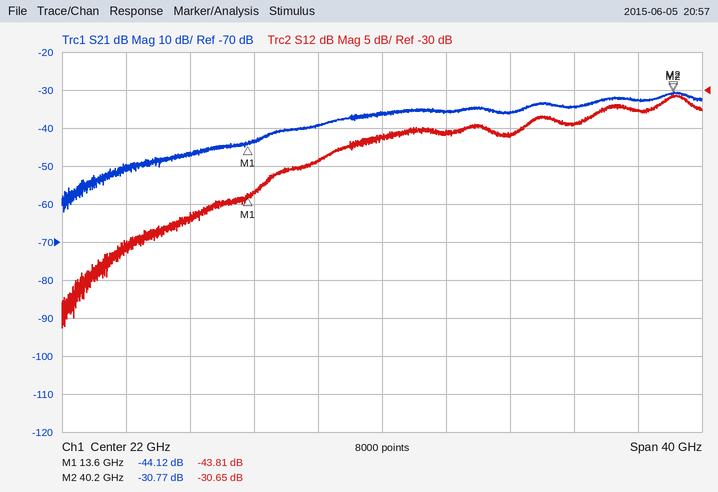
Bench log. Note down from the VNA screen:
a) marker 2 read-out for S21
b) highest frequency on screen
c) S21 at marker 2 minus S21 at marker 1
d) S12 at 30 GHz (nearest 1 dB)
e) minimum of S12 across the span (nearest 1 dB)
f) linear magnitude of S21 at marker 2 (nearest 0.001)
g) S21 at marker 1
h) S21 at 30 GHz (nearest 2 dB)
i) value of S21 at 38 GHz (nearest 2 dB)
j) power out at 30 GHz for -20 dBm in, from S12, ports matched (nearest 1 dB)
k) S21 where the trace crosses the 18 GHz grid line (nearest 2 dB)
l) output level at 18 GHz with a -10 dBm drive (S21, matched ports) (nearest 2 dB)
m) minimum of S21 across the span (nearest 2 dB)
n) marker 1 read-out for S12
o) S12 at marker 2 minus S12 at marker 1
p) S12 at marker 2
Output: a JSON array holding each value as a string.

["-30.77 dB", "42 GHz", "13.35 dB", "-36 dB", "-61 dB", "0.029", "-44.12 dB", "-36 dB", "-32 dB", "-56 dBm", "-40 dB", "-50 dBm", "-62 dB", "-43.81 dB", "13.16 dB", "-30.65 dB"]
